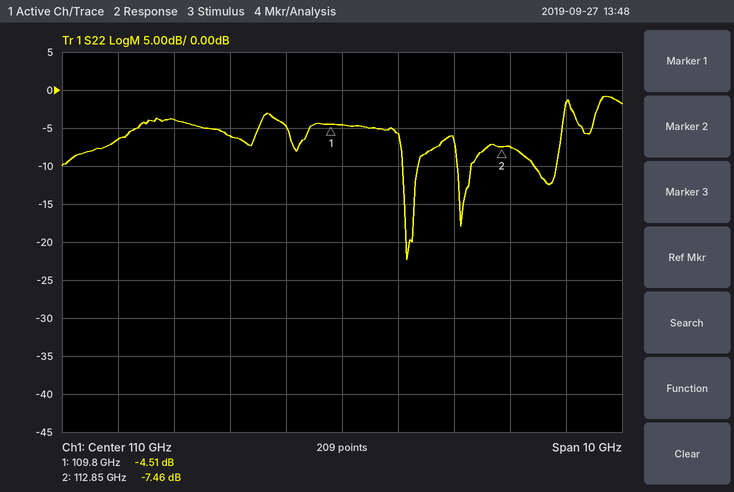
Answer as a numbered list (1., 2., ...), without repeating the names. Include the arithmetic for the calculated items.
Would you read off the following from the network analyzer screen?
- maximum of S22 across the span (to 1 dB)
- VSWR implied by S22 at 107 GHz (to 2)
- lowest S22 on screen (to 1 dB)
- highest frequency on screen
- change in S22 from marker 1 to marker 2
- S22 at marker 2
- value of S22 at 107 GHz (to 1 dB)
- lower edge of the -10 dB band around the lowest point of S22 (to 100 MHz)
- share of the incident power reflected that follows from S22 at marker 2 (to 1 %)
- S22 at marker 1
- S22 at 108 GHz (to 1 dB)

1. -1 dB
2. |Γ| = 10^(-4/20) = 0.6310; VSWR = (1 + 0.6310)/(1 − 0.6310) ≈ 4
3. -22 dB
4. 115 GHz
5. -7.46 − (-4.51) = -2.95 dB
6. -7.46 dB
7. -4 dB
8. 111.1 GHz
9. 10^(-7.46/10) ≈ 18 %
10. -4.51 dB
11. -6 dB
